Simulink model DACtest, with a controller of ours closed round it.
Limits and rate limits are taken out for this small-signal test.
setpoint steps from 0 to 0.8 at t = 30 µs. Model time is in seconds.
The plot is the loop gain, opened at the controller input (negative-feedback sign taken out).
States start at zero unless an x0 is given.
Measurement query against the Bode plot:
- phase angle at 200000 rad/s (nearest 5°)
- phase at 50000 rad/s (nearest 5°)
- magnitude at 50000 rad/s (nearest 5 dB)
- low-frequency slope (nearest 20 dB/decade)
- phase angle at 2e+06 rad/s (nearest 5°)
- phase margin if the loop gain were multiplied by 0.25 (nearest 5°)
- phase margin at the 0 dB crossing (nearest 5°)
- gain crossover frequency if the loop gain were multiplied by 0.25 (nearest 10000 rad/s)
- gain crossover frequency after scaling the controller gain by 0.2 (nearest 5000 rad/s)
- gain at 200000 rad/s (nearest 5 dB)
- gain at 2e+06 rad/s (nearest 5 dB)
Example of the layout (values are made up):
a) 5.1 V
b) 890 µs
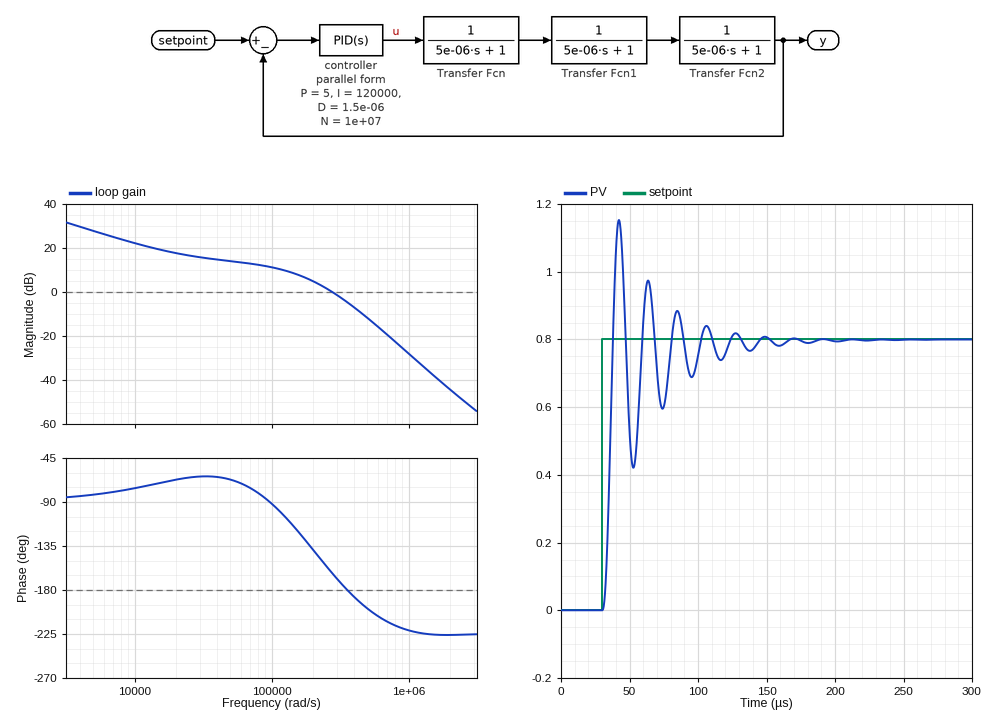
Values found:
a) -140°
b) -65°
c) 15 dB
d) -20 dB/decade
e) -225°
f) 95°
g) 15°
h) 90000 rad/s
i) 50000 rad/s
j) 5 dB
k) -45 dB
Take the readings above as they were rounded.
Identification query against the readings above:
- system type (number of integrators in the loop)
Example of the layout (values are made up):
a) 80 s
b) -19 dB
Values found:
a) 1
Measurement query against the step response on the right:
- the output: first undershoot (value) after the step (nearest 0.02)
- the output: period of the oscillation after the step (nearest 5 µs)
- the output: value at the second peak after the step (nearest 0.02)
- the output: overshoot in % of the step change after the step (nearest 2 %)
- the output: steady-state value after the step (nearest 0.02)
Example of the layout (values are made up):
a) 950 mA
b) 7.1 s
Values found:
a) 0.42
b) 20 µs
c) 0.98
d) 44 %
e) 0.80
